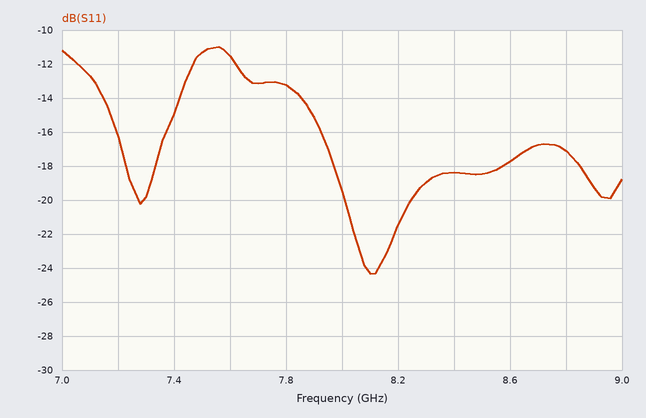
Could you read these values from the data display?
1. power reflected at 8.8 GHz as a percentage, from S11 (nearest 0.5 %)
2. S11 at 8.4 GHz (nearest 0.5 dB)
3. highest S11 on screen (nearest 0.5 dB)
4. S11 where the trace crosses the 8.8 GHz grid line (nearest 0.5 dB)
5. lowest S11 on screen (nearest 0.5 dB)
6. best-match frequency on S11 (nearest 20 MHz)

2.0 %
-18.5 dB
-11.0 dB
-17.0 dB
-24.5 dB
8.10 GHz
